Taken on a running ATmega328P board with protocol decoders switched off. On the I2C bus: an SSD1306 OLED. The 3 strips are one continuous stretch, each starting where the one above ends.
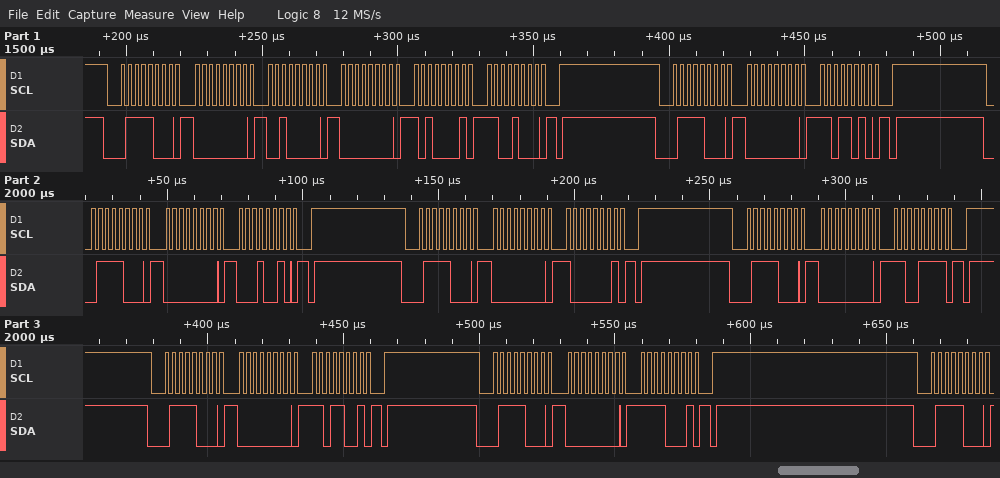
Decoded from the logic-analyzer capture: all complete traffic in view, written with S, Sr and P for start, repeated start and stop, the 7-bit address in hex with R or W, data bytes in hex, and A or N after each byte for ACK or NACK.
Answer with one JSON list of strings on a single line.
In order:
["S 3CW A 00 A 20 A 00 A A1 A C8 A P S 3CW A 00 A DA A P S 3CW A 00 A 12 A P S 3CW A 00 A 81 A P S 3CW A 00 A CF A P S 3CW A 00 A D9 A P S 3CW A 00 A F1 A P S 3CW A"]
